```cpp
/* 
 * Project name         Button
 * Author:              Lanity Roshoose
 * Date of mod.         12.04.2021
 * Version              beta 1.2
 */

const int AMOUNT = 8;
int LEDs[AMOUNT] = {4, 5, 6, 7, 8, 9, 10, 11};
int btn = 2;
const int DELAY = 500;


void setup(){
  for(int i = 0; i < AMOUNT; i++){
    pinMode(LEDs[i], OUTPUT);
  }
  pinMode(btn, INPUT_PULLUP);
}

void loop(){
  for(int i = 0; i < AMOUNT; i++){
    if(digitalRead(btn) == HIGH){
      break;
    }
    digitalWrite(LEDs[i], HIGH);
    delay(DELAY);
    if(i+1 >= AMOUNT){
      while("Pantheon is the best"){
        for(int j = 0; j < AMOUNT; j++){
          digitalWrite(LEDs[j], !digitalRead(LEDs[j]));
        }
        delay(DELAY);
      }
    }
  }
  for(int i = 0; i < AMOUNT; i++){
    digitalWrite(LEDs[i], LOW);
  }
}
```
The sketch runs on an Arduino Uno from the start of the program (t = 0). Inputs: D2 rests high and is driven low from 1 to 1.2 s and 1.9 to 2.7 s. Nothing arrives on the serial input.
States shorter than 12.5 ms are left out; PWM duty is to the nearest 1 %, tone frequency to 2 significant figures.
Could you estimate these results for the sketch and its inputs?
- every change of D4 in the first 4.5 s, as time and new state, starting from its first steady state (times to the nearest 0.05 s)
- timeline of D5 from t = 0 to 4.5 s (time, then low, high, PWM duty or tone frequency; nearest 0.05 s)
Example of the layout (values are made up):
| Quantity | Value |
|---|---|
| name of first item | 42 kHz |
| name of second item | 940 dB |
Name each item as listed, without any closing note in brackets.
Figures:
| Quantity | Value |
|---|---|
| every change of D4 in the first 4.5 s, as time and new state, starting from its first steady state | 0 s low; 1 s high; 1.5 s low; 1.9 s high; 2.9 s low |
| timeline of D5 from t = 0 to 4.5 s | 0 s low; 2.4 s high; 2.9 s low |
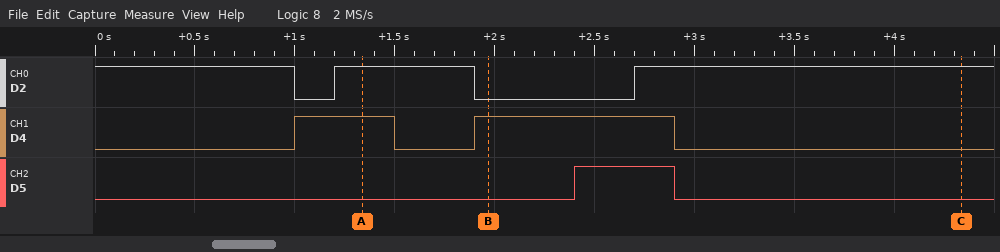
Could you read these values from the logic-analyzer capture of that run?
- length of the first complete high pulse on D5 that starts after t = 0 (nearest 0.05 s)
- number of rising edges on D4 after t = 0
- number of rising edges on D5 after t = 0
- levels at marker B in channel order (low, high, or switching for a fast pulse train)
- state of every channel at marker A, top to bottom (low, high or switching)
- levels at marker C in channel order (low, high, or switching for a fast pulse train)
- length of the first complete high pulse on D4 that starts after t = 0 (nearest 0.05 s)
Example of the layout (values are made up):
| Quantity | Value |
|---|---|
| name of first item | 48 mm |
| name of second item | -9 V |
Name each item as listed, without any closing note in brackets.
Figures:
| Quantity | Value |
|---|---|
| length of the first complete high pulse on D5 that starts after t = 0 | 0.50 s |
| number of rising edges on D4 after t = 0 | 2 |
| number of rising edges on D5 after t = 0 | 1 |
| levels at marker B in channel order | D2 low, D4 high, D5 low |
| state of every channel at marker A, top to bottom | D2 high, D4 high, D5 low |
| levels at marker C in channel order | D2 high, D4 low, D5 low |
| length of the first complete high pulse on D4 that starts after t = 0 | 0.50 s |
